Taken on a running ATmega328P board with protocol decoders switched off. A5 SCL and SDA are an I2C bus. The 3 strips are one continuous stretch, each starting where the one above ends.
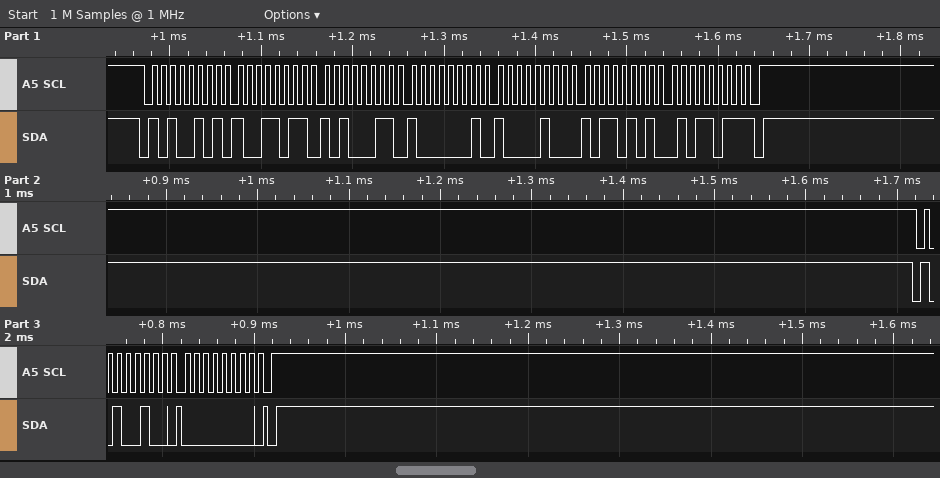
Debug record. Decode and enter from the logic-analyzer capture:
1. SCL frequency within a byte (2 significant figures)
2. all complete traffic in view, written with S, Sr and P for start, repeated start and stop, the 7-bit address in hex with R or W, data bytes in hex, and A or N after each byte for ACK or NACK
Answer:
100 kHz
S 52R A 9B A A3 A 81 A 84 A B5 A 5B N P S 52W A 00 A P
